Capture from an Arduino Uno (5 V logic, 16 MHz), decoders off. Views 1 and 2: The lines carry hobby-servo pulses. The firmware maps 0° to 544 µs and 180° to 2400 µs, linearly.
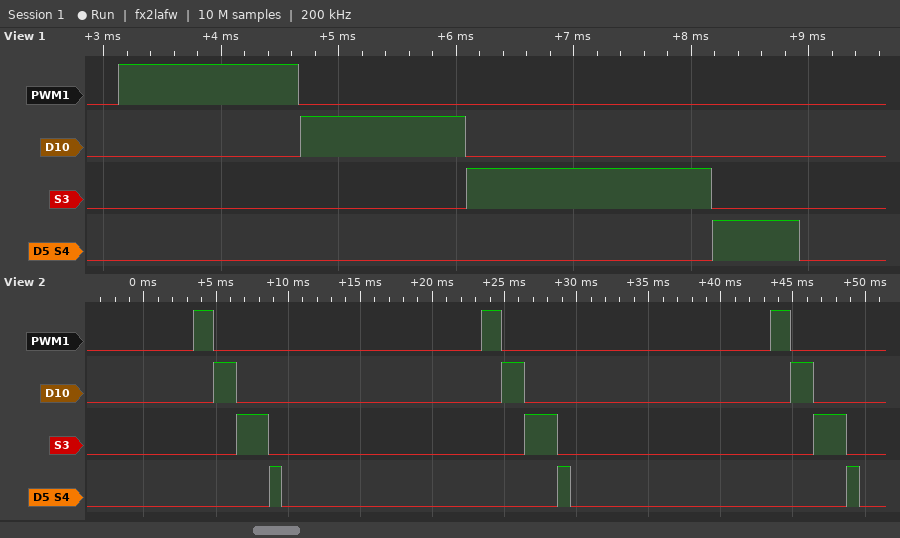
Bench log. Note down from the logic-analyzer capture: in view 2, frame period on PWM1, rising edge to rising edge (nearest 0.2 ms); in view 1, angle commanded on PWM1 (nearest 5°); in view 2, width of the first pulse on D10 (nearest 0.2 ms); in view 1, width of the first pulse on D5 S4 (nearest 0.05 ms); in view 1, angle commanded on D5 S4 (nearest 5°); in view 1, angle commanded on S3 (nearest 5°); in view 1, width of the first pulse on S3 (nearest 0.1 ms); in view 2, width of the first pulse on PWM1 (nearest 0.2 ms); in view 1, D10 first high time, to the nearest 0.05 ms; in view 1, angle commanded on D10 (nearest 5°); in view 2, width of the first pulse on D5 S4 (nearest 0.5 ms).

20.0 ms
95°
1.6 ms
0.75 ms
20°
150°
2.1 ms
1.4 ms
1.40 ms
85°
1.0 ms
